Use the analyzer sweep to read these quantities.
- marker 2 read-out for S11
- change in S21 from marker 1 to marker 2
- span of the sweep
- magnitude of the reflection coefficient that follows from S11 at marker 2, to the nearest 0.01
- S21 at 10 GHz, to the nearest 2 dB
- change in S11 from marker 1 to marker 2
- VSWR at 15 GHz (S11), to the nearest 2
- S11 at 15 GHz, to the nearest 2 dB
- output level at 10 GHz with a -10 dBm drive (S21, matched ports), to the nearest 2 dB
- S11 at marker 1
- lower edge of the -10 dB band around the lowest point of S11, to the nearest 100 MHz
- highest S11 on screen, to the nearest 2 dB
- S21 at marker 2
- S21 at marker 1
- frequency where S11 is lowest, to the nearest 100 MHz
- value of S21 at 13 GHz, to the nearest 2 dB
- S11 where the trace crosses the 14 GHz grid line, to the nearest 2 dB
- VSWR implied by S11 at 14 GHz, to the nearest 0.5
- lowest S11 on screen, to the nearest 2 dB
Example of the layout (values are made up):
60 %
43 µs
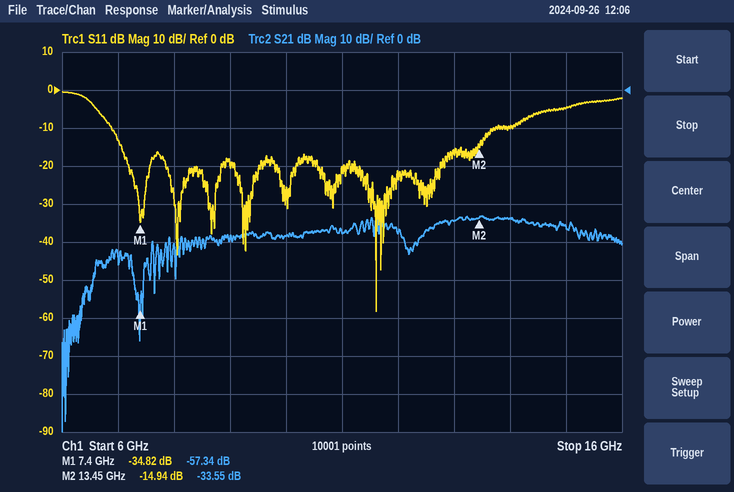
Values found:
-14.94 dB
23.79 dB
10 GHz
0.18
-38 dB
19.88 dB
4
-4 dB
-48 dBm
-34.82 dB
6.9 GHz
0 dB
-33.55 dB
-57.34 dB
11.6 GHz
-34 dB
-10 dB
2.0
-58 dB
